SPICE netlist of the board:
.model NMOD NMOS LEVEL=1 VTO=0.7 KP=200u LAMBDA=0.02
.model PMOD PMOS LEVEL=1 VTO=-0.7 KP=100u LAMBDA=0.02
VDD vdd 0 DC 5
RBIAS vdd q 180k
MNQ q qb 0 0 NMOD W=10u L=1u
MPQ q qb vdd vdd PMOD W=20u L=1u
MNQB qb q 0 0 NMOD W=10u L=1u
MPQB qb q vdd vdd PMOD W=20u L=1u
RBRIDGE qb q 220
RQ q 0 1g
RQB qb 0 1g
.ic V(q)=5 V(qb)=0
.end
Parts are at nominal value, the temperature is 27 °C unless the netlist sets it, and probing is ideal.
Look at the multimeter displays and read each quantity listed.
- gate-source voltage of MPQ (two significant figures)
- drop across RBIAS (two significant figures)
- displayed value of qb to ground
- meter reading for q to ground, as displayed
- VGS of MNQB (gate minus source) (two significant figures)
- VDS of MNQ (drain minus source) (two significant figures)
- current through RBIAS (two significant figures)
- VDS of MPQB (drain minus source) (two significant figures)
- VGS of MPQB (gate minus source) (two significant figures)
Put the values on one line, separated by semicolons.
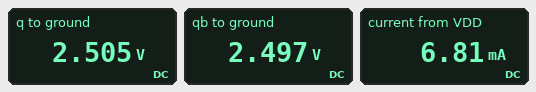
-2.5 V; 2.5 V; 2.497 V; 2.505 V; 2.5 V; 2.5 V; 14 µA; -2.5 V; -2.5 V
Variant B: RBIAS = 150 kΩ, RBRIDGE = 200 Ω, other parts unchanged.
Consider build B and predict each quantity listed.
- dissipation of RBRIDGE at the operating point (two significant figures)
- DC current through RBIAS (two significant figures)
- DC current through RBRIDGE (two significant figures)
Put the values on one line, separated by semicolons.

210 nW; 17 µA; 32 µA
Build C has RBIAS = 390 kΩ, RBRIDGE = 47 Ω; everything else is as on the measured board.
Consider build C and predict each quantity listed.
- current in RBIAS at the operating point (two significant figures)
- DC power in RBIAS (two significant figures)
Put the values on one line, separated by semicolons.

6.4 µA; 16 µW
